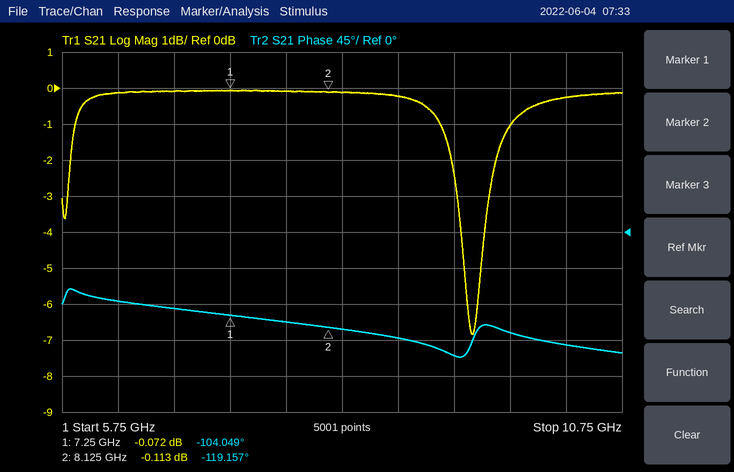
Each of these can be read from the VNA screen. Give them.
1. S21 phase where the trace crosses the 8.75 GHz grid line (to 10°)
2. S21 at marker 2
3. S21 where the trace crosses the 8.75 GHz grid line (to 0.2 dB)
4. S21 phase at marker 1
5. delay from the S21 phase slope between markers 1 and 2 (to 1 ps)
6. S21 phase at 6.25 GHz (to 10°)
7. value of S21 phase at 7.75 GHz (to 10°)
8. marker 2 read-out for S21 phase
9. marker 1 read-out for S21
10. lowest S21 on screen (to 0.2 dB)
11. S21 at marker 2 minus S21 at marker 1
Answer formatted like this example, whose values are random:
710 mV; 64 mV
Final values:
-130°; -0.113 dB; -0.2 dB; -104.049°; 48 ps; -90°; -110°; -119.157°; -0.072 dB; -6.8 dB; -0.041 dB
